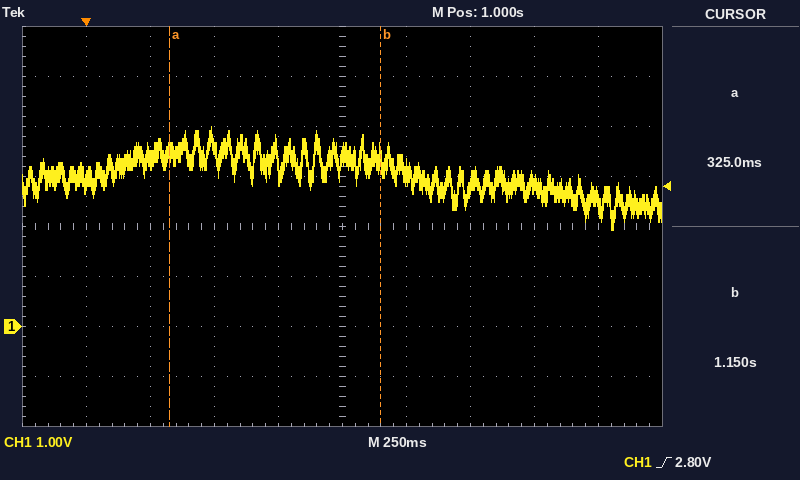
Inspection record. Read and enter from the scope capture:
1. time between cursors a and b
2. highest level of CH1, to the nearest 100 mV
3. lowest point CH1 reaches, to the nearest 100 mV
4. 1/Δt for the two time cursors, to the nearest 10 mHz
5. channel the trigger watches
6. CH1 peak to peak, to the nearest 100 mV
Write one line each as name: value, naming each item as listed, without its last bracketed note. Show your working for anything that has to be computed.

time between cursors a and b: 1.15 s − (325 ms) = 825 ms
highest level of CH1, to the nearest 100 mV: 4.0 V
lowest point CH1 reaches, to the nearest 100 mV: 1.9 V
1/Δt for the two time cursors, to the nearest 10 mHz: 1 / 825 ms ≈ 1.21 Hz
channel the trigger watches: CH1
CH1 peak to peak, to the nearest 100 mV: 4.0 V − (1.9 V) = 2.1 V
